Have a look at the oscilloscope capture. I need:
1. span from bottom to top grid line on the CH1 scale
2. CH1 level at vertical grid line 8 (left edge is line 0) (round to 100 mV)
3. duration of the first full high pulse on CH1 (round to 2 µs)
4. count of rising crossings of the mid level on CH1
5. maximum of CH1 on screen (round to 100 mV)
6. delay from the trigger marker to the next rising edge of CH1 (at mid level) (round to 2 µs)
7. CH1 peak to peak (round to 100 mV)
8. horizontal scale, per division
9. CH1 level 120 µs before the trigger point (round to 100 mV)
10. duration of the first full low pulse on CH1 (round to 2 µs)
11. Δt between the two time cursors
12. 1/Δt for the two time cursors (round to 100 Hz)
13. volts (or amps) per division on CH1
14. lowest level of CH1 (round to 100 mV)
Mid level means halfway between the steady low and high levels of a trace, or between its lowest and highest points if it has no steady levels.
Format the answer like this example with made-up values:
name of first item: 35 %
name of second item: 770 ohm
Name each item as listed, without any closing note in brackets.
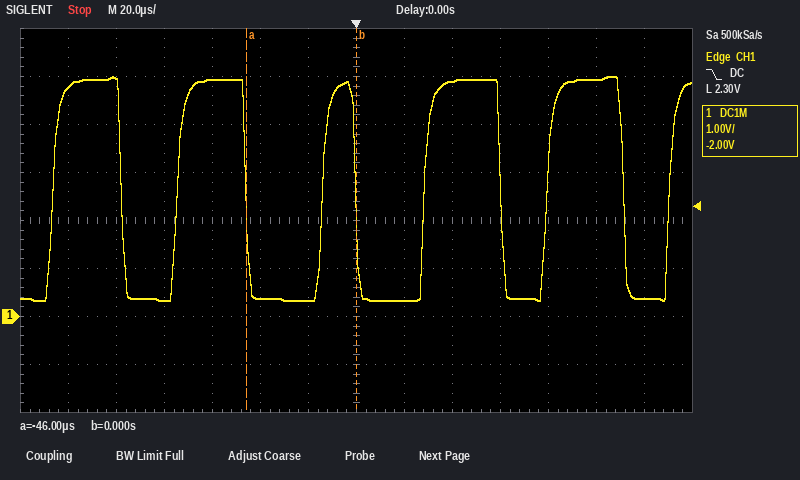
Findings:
span from bottom to top grid line on the CH1 scale: 8 V
CH1 level at vertical grid line 8 (left edge is line 0): 300 mV
duration of the first full high pulse on CH1: 28 µs
count of rising crossings of the mid level on CH1: 6
maximum of CH1 on screen: 5.0 V
delay from the trigger marker to the next rising edge of CH1 (at mid level): 28 µs
CH1 peak to peak: 4.7 V
horizontal scale, per division: 20 µs
CH1 level 120 µs before the trigger point: 4.8 V
duration of the first full low pulse on CH1: 24 µs
Δt between the two time cursors: 46 µs
1/Δt for the two time cursors: 21.7 kHz
volts (or amps) per division on CH1: 1 V
lowest level of CH1: 300 mV
